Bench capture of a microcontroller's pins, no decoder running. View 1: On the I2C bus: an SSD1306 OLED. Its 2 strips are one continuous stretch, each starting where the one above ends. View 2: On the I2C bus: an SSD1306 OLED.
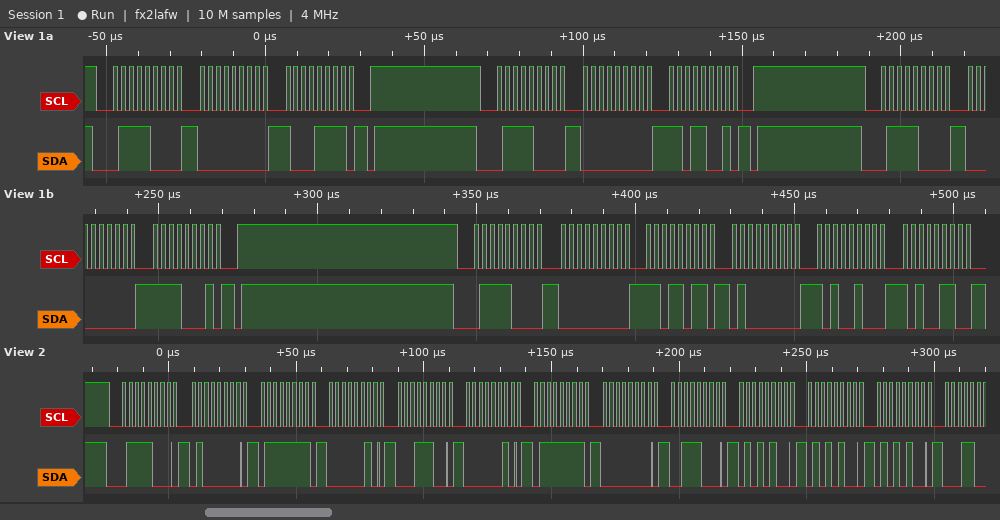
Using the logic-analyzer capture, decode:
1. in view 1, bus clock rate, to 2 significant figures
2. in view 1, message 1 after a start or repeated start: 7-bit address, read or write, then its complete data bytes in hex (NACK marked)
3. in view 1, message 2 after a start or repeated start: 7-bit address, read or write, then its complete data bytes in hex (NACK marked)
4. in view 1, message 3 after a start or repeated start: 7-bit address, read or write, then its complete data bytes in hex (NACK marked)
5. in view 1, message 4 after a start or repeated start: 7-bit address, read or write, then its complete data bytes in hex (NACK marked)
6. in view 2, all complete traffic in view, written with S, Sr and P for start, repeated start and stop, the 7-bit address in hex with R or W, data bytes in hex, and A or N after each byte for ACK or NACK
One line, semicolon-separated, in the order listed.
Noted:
400 kHz; 0x3C write: 00 8F; 0x3C write: 00 D9; 0x3C write: 00 F1; 0x3C write: 00 DB 40 A4 A6; S 3CW A 40 A 7F A 02 A 1C A 02 A 7F A 00 A 38 A 54 A 54 A 54 A
